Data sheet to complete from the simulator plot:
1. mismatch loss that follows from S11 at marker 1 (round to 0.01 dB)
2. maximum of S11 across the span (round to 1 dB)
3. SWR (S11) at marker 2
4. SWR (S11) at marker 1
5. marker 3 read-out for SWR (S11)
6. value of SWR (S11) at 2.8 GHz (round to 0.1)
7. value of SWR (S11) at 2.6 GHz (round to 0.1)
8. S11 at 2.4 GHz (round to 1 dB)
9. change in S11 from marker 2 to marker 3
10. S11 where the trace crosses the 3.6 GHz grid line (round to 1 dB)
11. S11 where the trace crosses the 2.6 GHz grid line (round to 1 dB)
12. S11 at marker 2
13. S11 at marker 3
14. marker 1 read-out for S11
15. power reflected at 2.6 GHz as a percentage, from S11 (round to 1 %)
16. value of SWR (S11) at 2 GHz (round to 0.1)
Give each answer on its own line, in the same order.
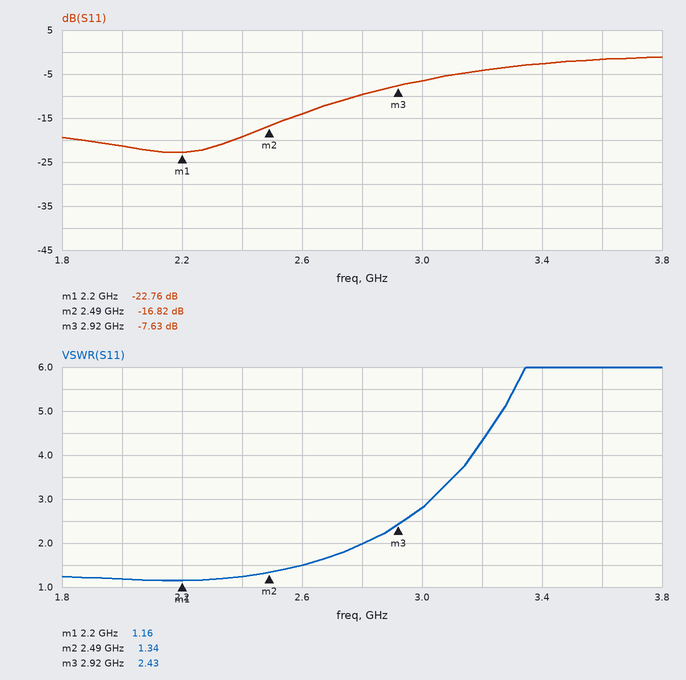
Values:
0.02 dB
-1 dB
1.34
1.16
2.43
2.0
1.5
-19 dB
9.19 dB
-2 dB
-14 dB
-16.82 dB
-7.63 dB
-22.76 dB
4 %
1.2
